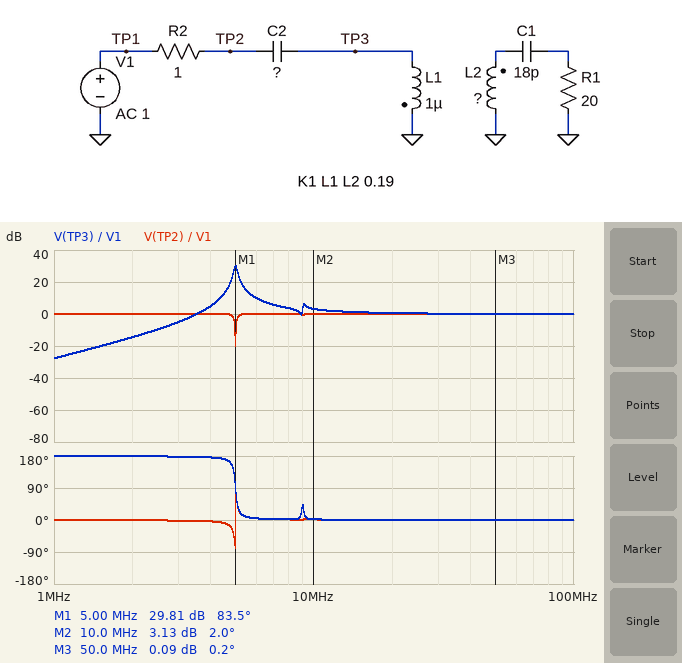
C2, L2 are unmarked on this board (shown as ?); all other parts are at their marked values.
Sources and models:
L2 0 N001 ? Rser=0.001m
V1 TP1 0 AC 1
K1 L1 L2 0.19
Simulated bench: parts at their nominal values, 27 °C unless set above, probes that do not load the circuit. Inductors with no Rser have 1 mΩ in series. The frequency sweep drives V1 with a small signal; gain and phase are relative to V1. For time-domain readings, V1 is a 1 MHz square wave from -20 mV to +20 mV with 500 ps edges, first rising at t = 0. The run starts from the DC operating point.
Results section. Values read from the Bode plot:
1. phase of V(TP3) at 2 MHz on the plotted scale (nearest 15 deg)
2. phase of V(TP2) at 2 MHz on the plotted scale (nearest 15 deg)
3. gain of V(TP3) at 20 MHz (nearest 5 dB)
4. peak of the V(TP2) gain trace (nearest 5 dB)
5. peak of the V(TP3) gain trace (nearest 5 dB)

180 deg
0 deg
0 dB
0 dB
30 dB
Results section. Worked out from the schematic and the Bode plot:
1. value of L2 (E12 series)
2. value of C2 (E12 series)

18 µH
1 nF
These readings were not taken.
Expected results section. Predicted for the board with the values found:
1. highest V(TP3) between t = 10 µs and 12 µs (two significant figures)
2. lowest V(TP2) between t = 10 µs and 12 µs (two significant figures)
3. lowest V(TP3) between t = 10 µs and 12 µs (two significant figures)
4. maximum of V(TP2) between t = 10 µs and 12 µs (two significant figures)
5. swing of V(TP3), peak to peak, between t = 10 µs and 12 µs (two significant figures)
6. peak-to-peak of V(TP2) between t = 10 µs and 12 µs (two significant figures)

180 mV
-25 mV
-180 mV
25 mV
360 mV
50 mV
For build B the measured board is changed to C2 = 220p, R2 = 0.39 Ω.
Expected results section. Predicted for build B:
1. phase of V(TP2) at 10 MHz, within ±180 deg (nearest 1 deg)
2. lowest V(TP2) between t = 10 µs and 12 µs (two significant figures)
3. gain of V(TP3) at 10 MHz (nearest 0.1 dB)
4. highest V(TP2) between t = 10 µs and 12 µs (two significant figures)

-1 deg
-20 mV
8.4 dB
20 mV
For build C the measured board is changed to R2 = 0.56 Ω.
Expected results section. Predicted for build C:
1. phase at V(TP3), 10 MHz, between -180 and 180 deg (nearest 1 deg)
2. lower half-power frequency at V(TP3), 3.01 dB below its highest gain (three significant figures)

1 deg
4.95 MHz
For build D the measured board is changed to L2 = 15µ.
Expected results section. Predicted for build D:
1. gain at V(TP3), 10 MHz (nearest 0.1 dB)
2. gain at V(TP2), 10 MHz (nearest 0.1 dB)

4.7 dB
-0.3 dB
